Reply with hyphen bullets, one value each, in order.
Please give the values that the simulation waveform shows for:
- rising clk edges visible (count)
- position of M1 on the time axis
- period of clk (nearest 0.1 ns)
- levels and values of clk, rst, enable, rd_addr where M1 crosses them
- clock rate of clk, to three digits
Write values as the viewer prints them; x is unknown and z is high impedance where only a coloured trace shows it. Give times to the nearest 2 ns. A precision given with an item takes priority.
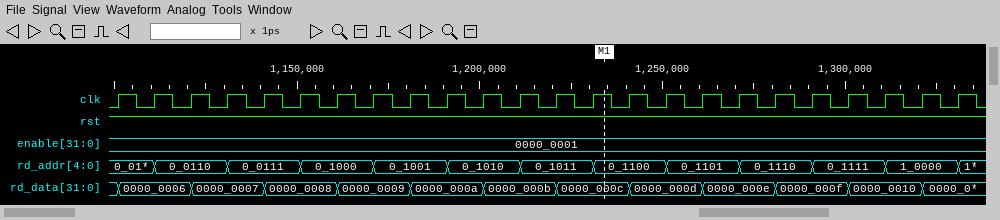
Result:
- 24
- 1234 ns
- 10 ns
- clk=1, rst=1, enable=0000_0001, rd_addr=0_1100
- 100 MHz
